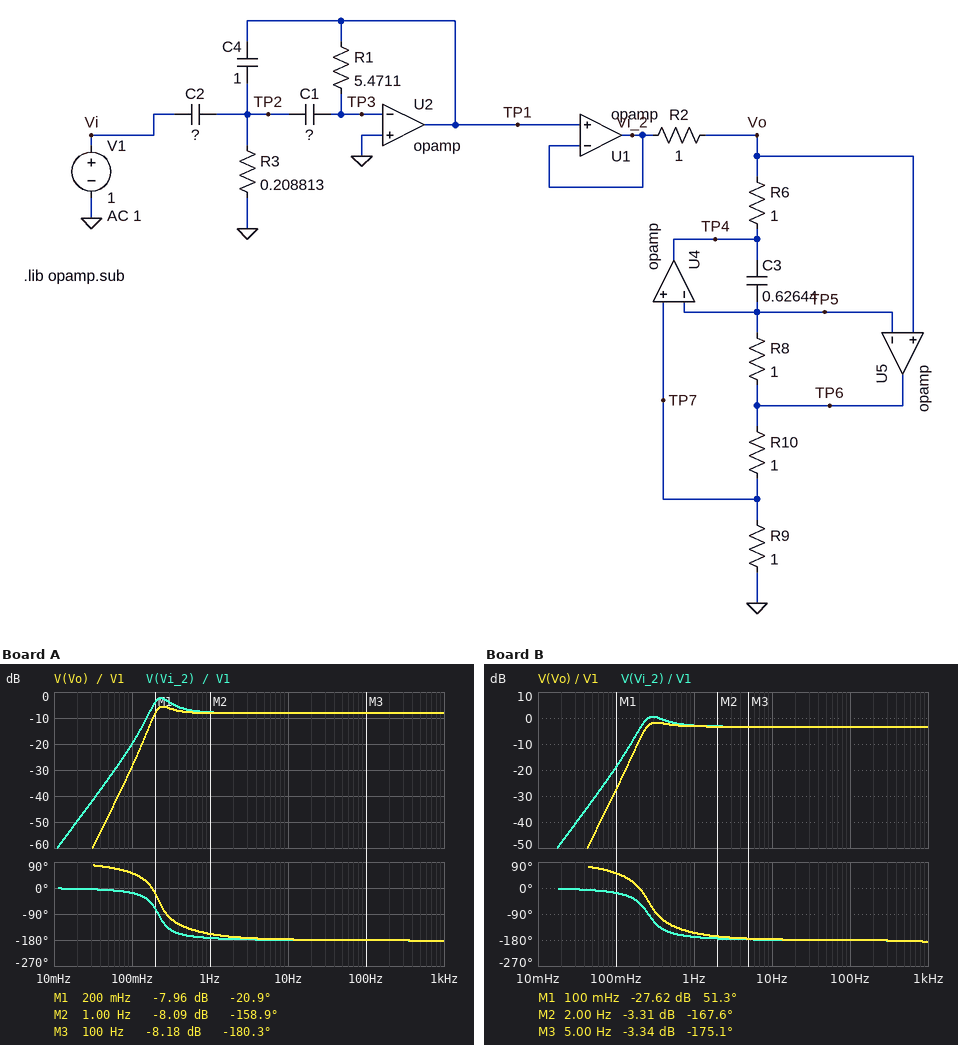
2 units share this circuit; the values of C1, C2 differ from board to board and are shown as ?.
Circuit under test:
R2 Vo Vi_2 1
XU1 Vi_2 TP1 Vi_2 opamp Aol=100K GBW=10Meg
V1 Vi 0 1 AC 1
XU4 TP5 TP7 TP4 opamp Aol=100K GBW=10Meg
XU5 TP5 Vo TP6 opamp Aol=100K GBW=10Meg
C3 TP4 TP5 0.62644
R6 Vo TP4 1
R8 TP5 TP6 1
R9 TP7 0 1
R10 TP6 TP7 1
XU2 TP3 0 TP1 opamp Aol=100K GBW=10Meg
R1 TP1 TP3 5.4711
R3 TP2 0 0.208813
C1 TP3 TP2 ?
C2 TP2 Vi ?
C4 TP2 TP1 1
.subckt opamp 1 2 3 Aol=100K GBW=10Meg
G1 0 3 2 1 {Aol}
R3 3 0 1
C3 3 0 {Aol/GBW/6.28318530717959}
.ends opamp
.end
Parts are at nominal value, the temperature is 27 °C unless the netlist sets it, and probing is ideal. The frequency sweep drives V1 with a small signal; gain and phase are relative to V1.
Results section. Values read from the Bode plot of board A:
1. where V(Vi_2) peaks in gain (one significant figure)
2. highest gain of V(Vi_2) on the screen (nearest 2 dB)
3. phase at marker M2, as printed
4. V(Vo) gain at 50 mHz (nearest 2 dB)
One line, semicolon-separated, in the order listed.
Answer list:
200 mHz; -2 dB; -158.9 deg; -48 dB
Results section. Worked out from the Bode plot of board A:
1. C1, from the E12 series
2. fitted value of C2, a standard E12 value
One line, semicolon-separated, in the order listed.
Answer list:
470 mF; 390 mF
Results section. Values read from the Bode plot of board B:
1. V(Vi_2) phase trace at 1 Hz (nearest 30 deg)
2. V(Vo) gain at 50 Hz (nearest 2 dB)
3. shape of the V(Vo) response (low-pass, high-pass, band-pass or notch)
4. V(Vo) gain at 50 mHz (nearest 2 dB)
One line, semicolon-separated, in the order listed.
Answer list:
-180 deg; -4 dB; high-pass; -46 dB
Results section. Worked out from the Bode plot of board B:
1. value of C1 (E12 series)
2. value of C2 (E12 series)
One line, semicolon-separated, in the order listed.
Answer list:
330 mF; 680 mF
